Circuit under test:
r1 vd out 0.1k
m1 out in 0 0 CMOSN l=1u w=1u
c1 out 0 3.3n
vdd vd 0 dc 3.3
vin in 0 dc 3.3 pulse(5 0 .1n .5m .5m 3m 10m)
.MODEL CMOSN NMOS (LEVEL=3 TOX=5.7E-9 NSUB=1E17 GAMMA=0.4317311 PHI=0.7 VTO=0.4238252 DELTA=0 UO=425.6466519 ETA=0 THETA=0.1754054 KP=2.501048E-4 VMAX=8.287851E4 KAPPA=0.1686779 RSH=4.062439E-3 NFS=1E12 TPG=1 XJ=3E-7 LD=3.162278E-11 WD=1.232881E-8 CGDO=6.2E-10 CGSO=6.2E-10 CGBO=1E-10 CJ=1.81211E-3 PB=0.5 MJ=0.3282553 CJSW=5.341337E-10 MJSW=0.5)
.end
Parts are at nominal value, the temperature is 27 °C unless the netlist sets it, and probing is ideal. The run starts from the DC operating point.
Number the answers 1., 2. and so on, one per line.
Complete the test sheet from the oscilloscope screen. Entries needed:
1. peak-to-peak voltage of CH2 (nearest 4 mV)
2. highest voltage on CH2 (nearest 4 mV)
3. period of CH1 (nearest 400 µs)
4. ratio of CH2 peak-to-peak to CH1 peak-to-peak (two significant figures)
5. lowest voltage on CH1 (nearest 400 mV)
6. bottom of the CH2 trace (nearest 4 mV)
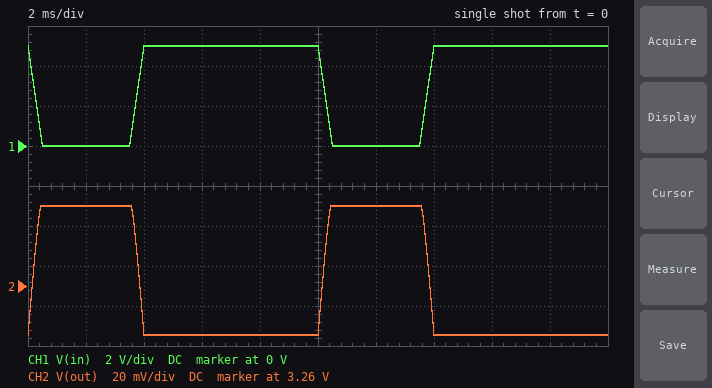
1. 64 mV
2. 3.300 V
3. 10.0 ms
4. 0.013
5. 0 V
6. 3.236 V
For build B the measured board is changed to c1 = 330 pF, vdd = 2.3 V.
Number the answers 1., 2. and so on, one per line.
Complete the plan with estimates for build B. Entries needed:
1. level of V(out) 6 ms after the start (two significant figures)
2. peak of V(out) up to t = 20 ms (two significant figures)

1. 2.2 V
2. 2.3 V
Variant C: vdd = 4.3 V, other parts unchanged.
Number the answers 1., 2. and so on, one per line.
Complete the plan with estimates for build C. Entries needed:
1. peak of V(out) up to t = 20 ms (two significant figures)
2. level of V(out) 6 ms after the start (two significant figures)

1. 4.3 V
2. 4.2 V
